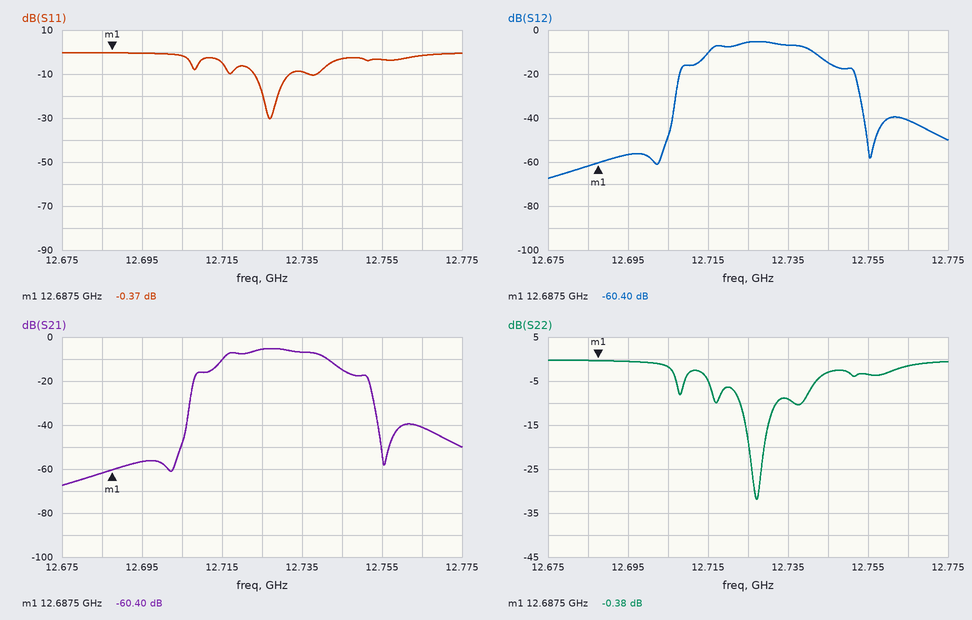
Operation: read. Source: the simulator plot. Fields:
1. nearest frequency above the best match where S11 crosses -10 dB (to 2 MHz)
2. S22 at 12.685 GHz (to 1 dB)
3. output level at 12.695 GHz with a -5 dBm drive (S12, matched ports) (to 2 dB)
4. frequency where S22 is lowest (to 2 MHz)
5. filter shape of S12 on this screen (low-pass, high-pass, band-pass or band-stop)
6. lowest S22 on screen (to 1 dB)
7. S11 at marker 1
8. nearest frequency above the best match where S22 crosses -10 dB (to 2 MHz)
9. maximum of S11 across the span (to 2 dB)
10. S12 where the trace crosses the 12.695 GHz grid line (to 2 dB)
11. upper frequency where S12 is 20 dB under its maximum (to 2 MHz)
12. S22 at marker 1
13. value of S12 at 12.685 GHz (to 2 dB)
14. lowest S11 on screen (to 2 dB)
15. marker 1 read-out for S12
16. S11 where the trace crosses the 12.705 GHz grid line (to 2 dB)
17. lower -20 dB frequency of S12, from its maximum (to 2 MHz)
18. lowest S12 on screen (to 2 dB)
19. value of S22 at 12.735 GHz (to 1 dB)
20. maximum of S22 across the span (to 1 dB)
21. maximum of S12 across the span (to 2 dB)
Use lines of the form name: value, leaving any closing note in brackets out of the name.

nearest frequency above the best match where S11 crosses -10 dB: 12.732 GHz
S22 at 12.685 GHz: 0 dB
output level at 12.695 GHz with a -5 dBm drive (S12, matched ports): -62 dBm
frequency where S22 is lowest: 12.728 GHz
filter shape of S12 on this screen: band-pass
lowest S22 on screen: -32 dB
S11 at marker 1: -0.37 dB
nearest frequency above the best match where S22 crosses -10 dB: 12.732 GHz
maximum of S11 across the span: 0 dB
S12 where the trace crosses the 12.695 GHz grid line: -56 dB
upper frequency where S12 is 20 dB under its maximum: 12.752 GHz
S22 at marker 1: -0.38 dB
value of S12 at 12.685 GHz: -62 dB
lowest S11 on screen: -30 dB
marker 1 read-out for S12: -60.40 dB
S11 where the trace crosses the 12.705 GHz grid line: -2 dB
lower -20 dB frequency of S12, from its maximum: 12.708 GHz
lowest S12 on screen: -68 dB
value of S22 at 12.735 GHz: -9 dB
maximum of S22 across the span: 0 dB
maximum of S12 across the span: -6 dB
